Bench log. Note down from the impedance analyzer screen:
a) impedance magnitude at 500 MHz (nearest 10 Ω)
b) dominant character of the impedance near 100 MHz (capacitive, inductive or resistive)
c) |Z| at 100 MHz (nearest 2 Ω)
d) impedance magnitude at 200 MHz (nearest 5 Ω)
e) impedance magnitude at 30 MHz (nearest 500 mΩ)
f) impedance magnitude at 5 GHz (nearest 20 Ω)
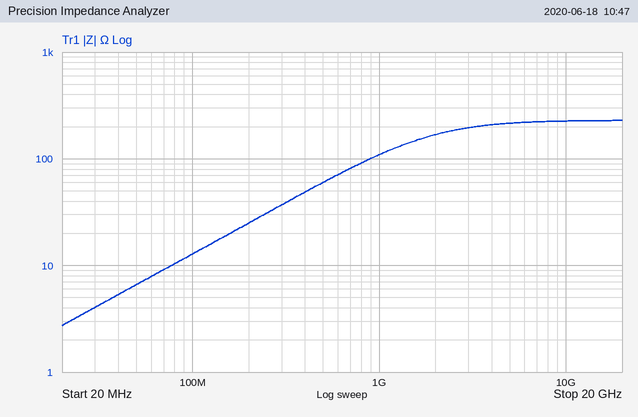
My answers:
60 Ω
inductive
12 Ω
25 Ω
4.0 Ω
220 Ω
